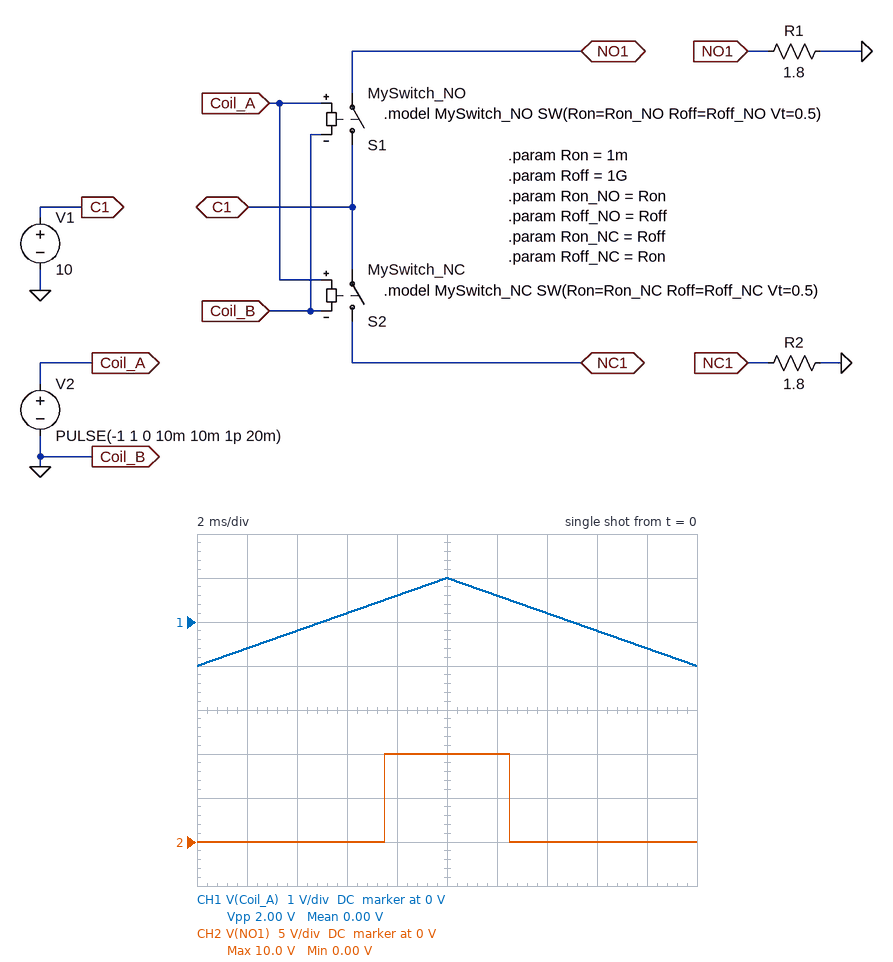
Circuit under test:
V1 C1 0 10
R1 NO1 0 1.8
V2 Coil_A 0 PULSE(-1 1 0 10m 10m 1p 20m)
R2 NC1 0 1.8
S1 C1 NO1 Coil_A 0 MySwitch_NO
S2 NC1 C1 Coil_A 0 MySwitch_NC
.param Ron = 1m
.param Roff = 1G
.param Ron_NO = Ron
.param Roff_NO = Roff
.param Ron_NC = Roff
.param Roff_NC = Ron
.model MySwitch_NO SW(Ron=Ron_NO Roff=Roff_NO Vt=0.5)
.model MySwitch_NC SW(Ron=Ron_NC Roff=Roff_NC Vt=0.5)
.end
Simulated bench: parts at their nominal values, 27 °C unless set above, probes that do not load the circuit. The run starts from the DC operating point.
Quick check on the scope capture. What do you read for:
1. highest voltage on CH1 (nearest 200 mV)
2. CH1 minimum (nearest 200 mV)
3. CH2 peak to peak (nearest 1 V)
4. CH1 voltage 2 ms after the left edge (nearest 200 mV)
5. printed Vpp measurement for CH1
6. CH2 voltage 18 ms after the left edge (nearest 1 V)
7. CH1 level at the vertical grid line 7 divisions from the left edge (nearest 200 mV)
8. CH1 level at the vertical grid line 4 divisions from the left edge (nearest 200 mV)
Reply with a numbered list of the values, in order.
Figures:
1. 1.0 V
2. -1.0 V
3. 10 V
4. -600 mV
5. 2.00 V
6. 0 V
7. 200 mV
8. 600 mV
